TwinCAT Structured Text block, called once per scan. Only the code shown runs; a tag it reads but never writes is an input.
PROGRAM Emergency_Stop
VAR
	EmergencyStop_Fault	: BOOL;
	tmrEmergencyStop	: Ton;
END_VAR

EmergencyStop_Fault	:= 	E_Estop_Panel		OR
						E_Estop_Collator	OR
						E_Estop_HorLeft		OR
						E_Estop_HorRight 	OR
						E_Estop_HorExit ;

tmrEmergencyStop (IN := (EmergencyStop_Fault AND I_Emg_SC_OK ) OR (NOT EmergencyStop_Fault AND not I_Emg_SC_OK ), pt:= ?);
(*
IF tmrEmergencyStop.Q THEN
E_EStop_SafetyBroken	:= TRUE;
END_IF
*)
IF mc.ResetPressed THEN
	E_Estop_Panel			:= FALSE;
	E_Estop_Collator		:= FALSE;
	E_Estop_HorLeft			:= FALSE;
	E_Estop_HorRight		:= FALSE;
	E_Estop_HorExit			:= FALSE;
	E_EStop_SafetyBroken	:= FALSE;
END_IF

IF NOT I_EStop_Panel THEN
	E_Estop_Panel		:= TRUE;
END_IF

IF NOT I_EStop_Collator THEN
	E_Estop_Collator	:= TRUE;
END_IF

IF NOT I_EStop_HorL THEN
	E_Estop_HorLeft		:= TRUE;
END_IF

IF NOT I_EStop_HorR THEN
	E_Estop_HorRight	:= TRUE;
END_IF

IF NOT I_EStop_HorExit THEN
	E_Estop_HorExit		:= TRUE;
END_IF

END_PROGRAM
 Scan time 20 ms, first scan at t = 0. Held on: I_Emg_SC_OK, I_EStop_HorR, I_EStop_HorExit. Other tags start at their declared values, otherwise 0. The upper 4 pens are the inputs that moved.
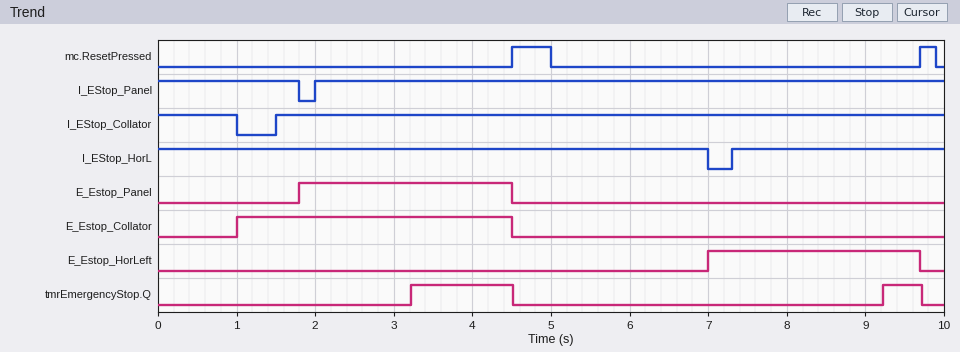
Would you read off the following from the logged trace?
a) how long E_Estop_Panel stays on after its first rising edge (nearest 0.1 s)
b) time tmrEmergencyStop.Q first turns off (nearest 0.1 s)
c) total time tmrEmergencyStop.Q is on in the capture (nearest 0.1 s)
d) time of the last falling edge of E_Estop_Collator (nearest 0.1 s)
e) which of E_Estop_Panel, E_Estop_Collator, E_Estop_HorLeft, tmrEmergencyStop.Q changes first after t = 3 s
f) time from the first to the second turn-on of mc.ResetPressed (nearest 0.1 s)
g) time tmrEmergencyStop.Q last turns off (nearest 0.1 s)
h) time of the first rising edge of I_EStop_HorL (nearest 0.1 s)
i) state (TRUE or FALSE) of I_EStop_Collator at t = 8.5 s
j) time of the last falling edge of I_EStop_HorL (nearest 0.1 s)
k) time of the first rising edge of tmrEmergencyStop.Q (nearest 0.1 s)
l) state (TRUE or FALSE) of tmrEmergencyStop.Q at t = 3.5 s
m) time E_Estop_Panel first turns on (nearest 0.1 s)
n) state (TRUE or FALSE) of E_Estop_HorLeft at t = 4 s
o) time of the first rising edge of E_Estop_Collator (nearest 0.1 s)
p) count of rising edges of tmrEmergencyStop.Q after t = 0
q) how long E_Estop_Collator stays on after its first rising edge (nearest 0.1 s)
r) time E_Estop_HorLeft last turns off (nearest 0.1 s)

2.7 s
4.5 s
1.8 s
4.5 s
tmrEmergencyStop.Q
5.2 s
9.7 s
7.3 s
TRUE
7.0 s
3.2 s
TRUE
1.8 s
FALSE
1.0 s
2
3.5 s
9.7 s
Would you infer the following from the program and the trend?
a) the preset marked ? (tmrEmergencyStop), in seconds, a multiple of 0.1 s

2.2 s
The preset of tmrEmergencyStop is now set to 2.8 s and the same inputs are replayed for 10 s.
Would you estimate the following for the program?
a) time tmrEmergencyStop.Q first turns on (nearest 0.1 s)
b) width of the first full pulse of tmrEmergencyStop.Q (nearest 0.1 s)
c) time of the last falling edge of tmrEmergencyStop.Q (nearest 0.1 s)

3.8 s
0.7 s
4.5 s
